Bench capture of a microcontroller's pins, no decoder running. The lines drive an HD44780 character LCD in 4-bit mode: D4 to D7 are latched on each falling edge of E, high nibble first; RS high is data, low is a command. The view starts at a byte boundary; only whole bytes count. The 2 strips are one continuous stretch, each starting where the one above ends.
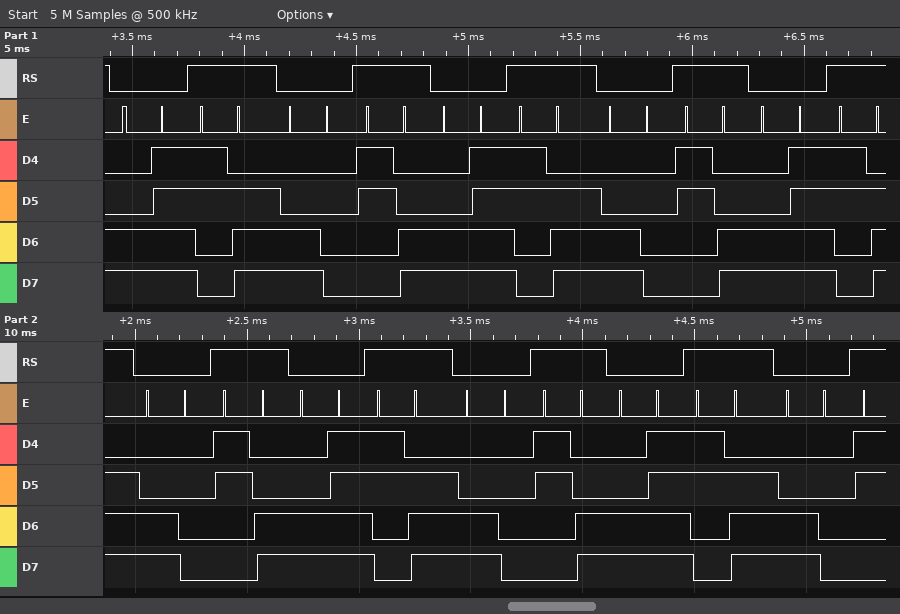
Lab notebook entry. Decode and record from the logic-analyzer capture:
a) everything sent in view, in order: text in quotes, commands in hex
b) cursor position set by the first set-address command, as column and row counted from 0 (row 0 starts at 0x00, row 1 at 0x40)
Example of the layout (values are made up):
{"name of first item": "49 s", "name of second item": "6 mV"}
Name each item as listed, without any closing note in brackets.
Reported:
{"everything sent in view, in order: text in quotes, commands in hex": "0xCF \">\" 0xC0 \"<\" 0xCF \">\" 0xC0 \"<\" 0xCF \">\" 0xC0 \"<\" 0xCF \">\" 0xC0 \"<\" 0xCF \">\" 0xC0", "cursor position set by the first set-address command, as column and row counted from 0": "column 15, row 1"}
